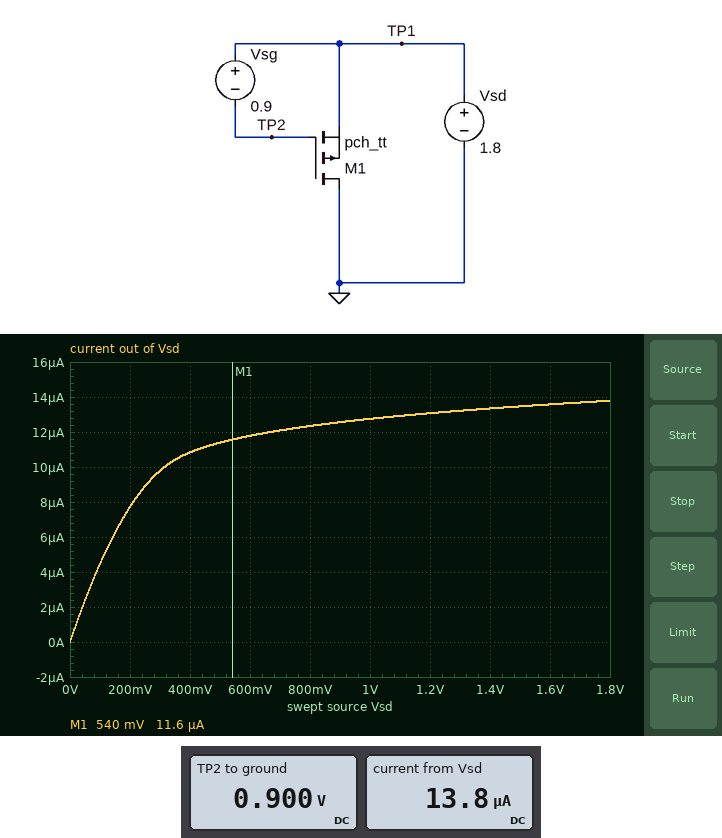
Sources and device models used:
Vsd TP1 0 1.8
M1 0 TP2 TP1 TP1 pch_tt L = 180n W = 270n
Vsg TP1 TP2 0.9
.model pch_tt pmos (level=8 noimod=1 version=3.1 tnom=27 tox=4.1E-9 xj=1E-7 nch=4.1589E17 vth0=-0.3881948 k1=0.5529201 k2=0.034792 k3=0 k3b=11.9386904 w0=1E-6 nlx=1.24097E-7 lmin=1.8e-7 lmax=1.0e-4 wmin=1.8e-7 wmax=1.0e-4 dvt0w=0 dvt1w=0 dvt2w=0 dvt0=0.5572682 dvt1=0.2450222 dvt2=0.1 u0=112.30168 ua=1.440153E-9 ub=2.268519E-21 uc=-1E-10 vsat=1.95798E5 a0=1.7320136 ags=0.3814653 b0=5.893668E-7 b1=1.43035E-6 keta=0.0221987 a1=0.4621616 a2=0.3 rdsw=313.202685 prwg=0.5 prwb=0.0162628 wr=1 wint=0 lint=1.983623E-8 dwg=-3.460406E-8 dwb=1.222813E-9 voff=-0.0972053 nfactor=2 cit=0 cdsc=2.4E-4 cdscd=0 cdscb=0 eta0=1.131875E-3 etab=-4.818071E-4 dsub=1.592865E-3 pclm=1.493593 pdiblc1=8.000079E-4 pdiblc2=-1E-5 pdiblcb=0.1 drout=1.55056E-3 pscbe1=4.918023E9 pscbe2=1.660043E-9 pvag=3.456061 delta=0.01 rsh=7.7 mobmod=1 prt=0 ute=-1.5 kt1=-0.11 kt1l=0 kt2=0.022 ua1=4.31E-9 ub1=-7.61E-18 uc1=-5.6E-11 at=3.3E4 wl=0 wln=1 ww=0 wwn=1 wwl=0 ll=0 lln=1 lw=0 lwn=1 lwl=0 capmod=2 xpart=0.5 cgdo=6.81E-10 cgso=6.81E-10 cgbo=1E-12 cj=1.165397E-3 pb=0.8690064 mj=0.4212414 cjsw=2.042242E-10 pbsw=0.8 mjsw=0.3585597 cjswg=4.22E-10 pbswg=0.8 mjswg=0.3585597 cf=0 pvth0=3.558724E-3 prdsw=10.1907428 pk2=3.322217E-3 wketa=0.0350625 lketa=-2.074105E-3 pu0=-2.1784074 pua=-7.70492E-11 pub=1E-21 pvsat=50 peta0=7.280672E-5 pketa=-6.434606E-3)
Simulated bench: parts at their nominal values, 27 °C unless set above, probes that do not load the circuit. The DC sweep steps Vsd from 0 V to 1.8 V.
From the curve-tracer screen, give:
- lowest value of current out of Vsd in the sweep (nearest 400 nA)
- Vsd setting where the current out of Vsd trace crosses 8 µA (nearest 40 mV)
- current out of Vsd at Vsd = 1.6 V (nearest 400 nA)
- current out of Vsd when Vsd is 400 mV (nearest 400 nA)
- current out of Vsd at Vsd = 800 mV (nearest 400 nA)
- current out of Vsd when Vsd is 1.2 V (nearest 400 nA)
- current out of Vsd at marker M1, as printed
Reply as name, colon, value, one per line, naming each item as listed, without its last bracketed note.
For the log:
lowest value of current out of Vsd in the sweep: 0 A
Vsd setting where the current out of Vsd trace crosses 8 µA: 200 mV
current out of Vsd at Vsd = 1.6 V: 13.6 µA
current out of Vsd when Vsd is 400 mV: 10.8 µA
current out of Vsd at Vsd = 800 mV: 12.4 µA
current out of Vsd when Vsd is 1.2 V: 13.2 µA
current out of Vsd at marker M1, as printed: 11.6 µA
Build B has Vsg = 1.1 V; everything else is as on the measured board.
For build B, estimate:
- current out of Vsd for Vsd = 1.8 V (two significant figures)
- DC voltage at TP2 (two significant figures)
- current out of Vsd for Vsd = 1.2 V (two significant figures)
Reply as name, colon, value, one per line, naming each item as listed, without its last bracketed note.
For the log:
current out of Vsd for Vsd = 1.8 V: 26 µA
DC voltage at TP2: 700 mV
current out of Vsd for Vsd = 1.2 V: 25 µA
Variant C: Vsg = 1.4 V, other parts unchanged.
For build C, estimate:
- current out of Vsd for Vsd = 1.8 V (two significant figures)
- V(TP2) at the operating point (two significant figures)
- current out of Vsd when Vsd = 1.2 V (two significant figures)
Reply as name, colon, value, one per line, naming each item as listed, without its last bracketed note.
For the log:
current out of Vsd for Vsd = 1.8 V: 50 µA
V(TP2) at the operating point: 400 mV
current out of Vsd when Vsd = 1.2 V: 48 µA
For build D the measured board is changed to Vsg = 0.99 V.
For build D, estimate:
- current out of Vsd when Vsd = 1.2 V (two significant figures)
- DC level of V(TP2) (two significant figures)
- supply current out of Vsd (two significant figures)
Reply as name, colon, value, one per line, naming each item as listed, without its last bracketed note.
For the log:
current out of Vsd when Vsd = 1.2 V: 18 µA
DC level of V(TP2): 810 mV
supply current out of Vsd: 19 µA
